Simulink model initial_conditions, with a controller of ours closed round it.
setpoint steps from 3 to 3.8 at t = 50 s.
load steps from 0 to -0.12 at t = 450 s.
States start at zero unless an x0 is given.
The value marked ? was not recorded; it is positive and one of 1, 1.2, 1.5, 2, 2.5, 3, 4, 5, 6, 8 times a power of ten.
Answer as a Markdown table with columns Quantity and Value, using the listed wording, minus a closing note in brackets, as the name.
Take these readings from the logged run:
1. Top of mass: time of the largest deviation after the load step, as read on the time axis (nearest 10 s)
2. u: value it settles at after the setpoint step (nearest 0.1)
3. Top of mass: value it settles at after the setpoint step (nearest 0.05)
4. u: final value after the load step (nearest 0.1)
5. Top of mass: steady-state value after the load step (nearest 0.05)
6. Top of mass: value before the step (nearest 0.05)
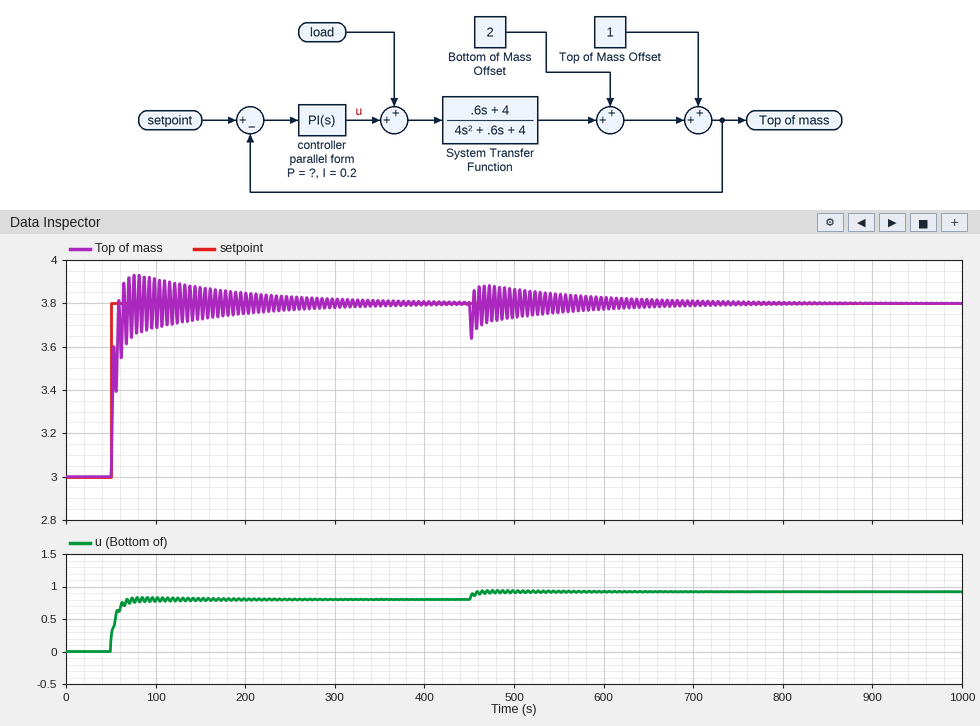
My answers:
| Quantity | Value |
|---|---|
| Top of mass: time of the largest deviation after the load step, as read on the time axis | 450 s |
| u: value it settles at after the setpoint step | 0.8 |
| Top of mass: value it settles at after the setpoint step | 3.80 |
| u: final value after the load step | 0.9 |
| Top of mass: steady-state value after the load step | 3.80 |
| Top of mass: value before the step | 3.00 |
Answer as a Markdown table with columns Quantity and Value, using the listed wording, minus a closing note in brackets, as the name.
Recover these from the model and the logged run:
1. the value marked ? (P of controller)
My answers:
| Quantity | Value |
|---|---|
| the value marked ? | 0.2 |
